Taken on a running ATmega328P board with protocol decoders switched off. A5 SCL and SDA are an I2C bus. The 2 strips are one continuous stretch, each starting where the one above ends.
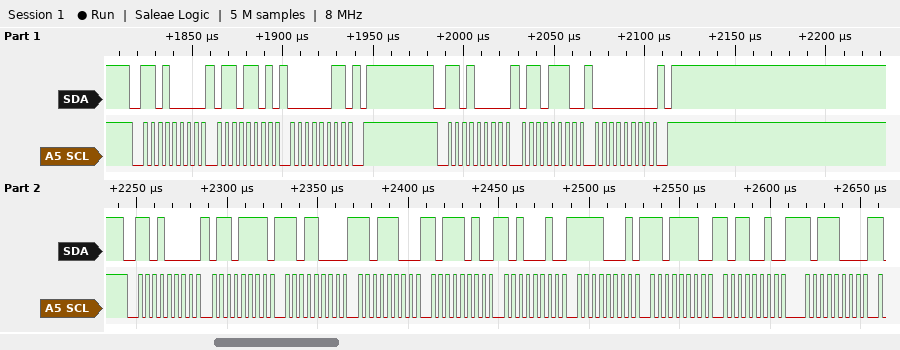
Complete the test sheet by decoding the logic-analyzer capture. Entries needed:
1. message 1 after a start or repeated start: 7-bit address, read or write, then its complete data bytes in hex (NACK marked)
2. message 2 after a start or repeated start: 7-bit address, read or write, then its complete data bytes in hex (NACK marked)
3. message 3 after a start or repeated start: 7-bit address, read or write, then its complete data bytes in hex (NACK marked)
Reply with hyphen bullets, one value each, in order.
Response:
- 0x68 write: 6D 03
- 0x68 write: 6E 00
- 0x68 write: 6F D8 DC BA A2 F1 DE B2 B8
